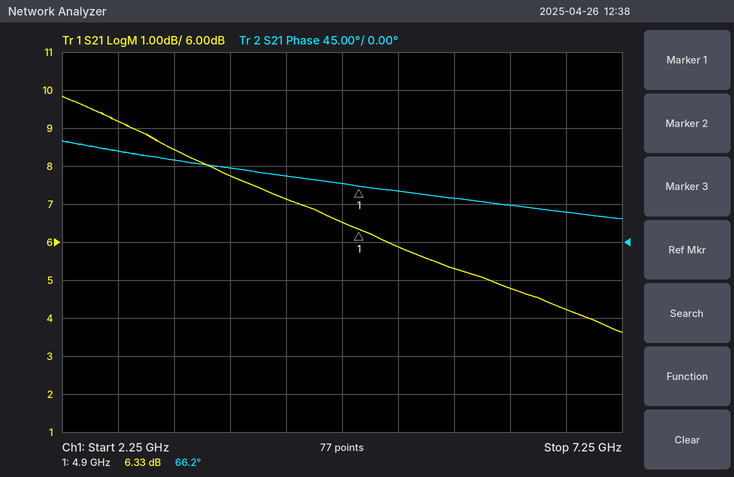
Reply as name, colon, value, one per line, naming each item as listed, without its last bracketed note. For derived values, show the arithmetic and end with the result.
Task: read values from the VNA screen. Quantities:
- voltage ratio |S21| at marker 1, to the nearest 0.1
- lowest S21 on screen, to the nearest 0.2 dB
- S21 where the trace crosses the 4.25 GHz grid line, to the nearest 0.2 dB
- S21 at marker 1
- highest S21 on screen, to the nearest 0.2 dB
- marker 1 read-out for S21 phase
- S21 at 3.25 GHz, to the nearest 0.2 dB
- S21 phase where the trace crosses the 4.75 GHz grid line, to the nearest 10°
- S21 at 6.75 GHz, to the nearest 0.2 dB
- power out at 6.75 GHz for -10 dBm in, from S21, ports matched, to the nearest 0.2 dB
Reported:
voltage ratio |S21| at marker 1, to the nearest 0.1: 10^(6.33/20) ≈ 2.1
lowest S21 on screen, to the nearest 0.2 dB: 3.6 dB
S21 where the trace crosses the 4.25 GHz grid line, to the nearest 0.2 dB: 7.2 dB
S21 at marker 1: 6.33 dB
highest S21 on screen, to the nearest 0.2 dB: 9.8 dB
marker 1 read-out for S21 phase: 66.2°
S21 at 3.25 GHz, to the nearest 0.2 dB: 8.4 dB
S21 phase where the trace crosses the 4.75 GHz grid line, to the nearest 10°: 70°
S21 at 6.75 GHz, to the nearest 0.2 dB: 4.2 dB
power out at 6.75 GHz for -10 dBm in, from S21, ports matched, to the nearest 0.2 dB: -10 dBm + (4.2 dB) = -5.8 dBm
